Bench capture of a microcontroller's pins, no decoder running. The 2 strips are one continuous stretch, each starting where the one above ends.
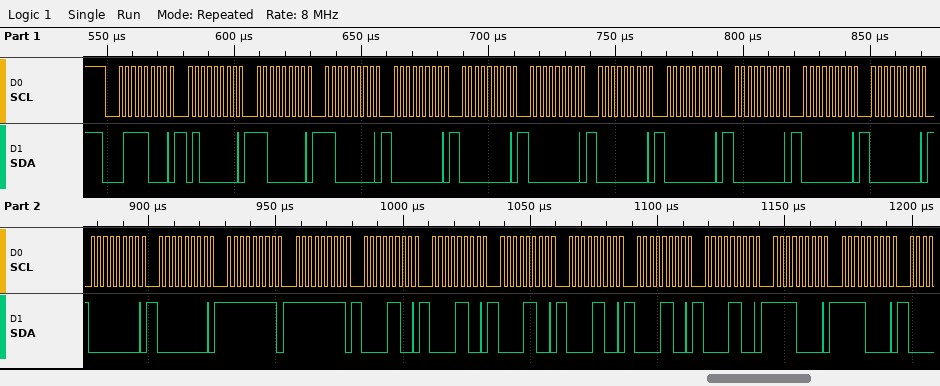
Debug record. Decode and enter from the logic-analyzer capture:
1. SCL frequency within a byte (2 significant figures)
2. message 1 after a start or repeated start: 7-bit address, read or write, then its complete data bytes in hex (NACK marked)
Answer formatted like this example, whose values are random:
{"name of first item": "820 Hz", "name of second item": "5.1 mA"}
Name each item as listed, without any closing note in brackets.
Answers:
{"SCL frequency within a byte": "400 kHz", "message 1 after a start or repeated start: 7-bit address, read or write, then its complete data bytes in hex": "0x3C write: 40 C0 C0 00 00 00 00 00 00 00 00 00 00 FF FF 0C 0C 0C 0C 0C 0C F0 F0"}
